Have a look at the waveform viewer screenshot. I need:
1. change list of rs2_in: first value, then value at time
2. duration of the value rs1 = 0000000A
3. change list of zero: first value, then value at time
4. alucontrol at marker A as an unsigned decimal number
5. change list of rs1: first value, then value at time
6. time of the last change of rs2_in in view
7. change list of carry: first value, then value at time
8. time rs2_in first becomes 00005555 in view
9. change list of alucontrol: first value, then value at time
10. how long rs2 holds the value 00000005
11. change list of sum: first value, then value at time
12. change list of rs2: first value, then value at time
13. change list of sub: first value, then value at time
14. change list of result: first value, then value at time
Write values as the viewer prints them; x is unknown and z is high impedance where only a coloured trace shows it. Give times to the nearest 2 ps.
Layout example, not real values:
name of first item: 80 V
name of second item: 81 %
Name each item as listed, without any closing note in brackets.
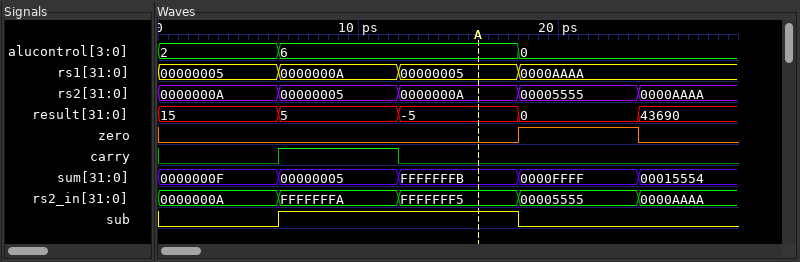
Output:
change list of rs2_in: first value, then value at time: 0000000A, FFFFFFFA at 6 ps, FFFFFFF5 at 12 ps, 00005555 at 18 ps, 0000AAAA at 24 ps
duration of the value rs1 = 0000000A: 6 ps
change list of zero: first value, then value at time: 0, 1 at 18 ps, 0 at 24 ps
alucontrol at marker A as an unsigned decimal number: 6
change list of rs1: first value, then value at time: 00000005, 0000000A at 6 ps, 00000005 at 12 ps, 0000AAAA at 18 ps
time of the last change of rs2_in in view: 24 ps
change list of carry: first value, then value at time: 0, 1 at 6 ps, 0 at 12 ps
time rs2_in first becomes 00005555 in view: 18 ps
change list of alucontrol: first value, then value at time: 2, 6 at 6 ps, 0 at 18 ps
how long rs2 holds the value 00000005: 6 ps
change list of sum: first value, then value at time: 0000000F, 00000005 at 6 ps, FFFFFFFB at 12 ps, 0000FFFF at 18 ps, 00015554 at 24 ps
change list of rs2: first value, then value at time: 0000000A, 00000005 at 6 ps, 0000000A at 12 ps, 00005555 at 18 ps, 0000AAAA at 24 ps
change list of sub: first value, then value at time: 0, 1 at 6 ps, 0 at 18 ps
change list of result: first value, then value at time: 15, 5 at 6 ps, -5 at 12 ps, 0 at 18 ps, 43690 at 24 ps
